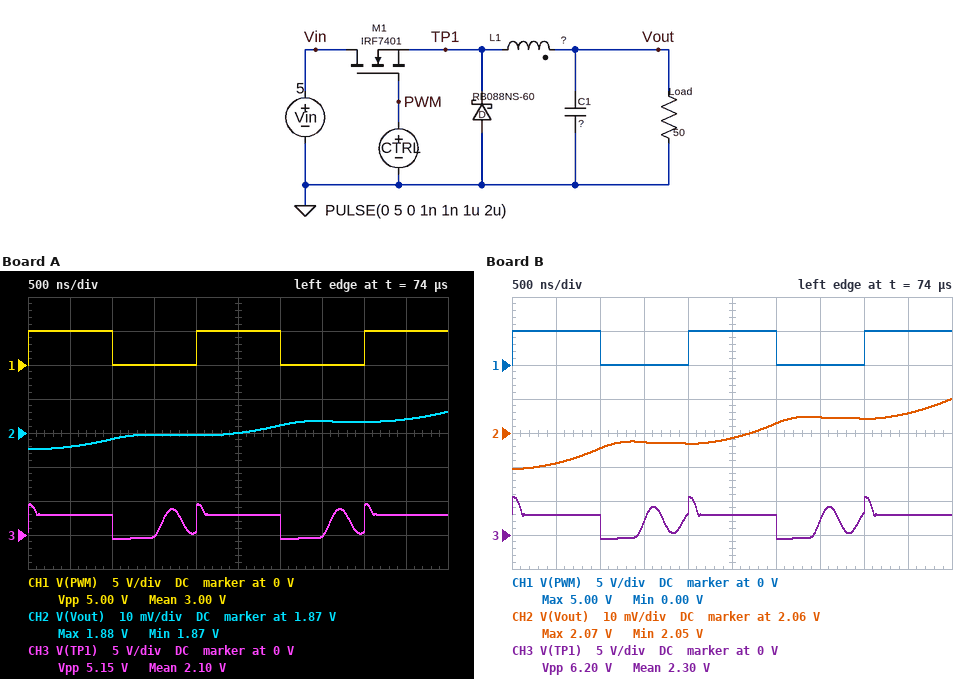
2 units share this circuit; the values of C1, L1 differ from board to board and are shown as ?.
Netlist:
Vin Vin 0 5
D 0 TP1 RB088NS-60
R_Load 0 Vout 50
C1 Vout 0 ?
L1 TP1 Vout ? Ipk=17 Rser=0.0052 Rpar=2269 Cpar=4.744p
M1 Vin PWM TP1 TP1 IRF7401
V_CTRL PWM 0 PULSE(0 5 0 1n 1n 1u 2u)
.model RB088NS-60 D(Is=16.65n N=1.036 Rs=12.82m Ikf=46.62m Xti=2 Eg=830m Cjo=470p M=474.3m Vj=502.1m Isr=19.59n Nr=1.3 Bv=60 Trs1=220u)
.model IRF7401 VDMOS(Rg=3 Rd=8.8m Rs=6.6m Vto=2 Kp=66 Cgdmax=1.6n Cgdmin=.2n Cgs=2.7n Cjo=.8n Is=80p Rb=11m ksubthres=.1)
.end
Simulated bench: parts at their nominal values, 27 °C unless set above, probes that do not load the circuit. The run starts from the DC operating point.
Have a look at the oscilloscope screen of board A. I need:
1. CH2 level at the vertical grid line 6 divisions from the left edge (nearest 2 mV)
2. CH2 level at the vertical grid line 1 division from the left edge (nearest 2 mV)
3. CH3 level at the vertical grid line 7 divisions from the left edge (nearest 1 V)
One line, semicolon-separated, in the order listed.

1.872 V; 1.866 V; 0 V
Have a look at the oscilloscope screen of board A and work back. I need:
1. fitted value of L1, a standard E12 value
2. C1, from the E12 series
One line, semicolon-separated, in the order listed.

1.8 µH; 100 µF
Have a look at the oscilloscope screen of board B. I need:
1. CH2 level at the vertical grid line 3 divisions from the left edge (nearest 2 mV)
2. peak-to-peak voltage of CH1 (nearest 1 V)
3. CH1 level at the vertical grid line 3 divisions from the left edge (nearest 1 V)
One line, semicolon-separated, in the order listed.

2.058 V; 5 V; 0 V
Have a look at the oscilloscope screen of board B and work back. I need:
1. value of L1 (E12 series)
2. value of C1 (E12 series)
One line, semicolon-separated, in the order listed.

1.5 µH; 56 µF
